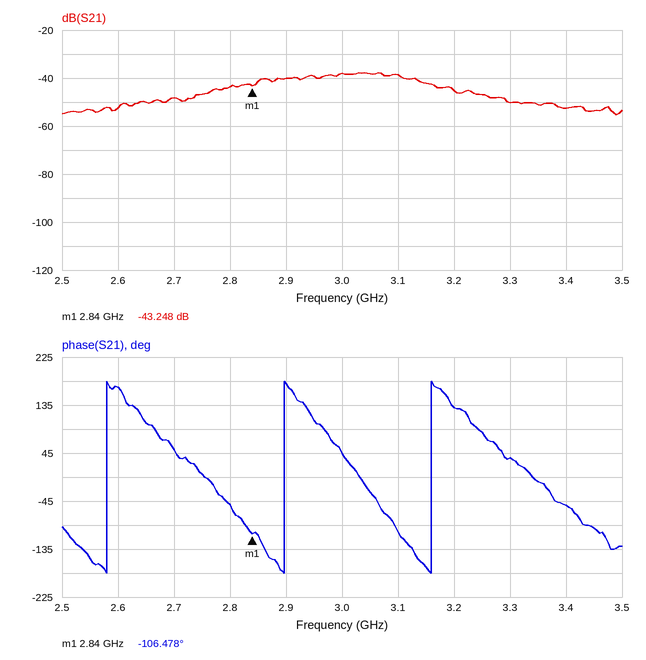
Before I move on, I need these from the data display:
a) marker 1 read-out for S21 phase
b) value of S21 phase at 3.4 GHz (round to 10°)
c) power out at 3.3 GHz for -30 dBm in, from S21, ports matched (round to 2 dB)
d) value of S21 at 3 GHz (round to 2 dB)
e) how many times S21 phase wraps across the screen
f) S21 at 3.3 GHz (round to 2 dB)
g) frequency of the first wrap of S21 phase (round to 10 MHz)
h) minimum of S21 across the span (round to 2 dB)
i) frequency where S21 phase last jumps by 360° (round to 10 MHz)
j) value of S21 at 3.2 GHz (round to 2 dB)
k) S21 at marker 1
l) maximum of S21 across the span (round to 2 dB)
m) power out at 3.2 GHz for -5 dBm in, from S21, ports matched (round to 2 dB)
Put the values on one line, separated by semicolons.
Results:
-106.478°; -50°; -80 dBm; -38 dB; 3; -50 dB; 2.58 GHz; -56 dB; 3.16 GHz; -46 dB; -43.248 dB; -38 dB; -50 dBm
